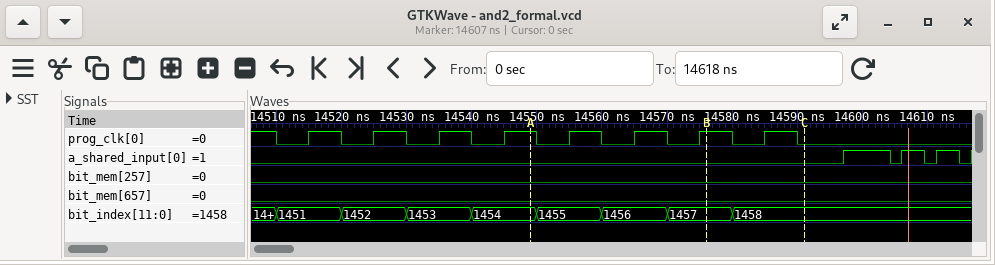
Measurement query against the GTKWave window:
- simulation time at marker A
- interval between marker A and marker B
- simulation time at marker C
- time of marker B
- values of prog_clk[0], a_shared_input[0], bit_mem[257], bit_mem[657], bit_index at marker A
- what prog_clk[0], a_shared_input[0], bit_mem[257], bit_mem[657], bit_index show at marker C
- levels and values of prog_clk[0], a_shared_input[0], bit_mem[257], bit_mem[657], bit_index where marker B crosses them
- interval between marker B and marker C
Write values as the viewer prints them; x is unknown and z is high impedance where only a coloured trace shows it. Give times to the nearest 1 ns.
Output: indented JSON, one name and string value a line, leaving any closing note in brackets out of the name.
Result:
{
  "simulation time at marker A": "14549 ns",
  "interval between marker A and marker B": "27 ns",
  "simulation time at marker C": "14591 ns",
  "time of marker B": "14576 ns",
  "values of prog_clk[0], a_shared_input[0], bit_mem[257], bit_mem[657], bit_index at marker A": "prog_clk[0]=1, a_shared_input[0]=0, bit_mem[257]=0, bit_mem[657]=0, bit_index=1454",
  "what prog_clk[0], a_shared_input[0], bit_mem[257], bit_mem[657], bit_index show at marker C": "prog_clk[0]=0, a_shared_input[0]=0, bit_mem[257]=0, bit_mem[657]=0, bit_index=1458",
  "levels and values of prog_clk[0], a_shared_input[0], bit_mem[257], bit_mem[657], bit_index where marker B crosses them": "prog_clk[0]=1, a_shared_input[0]=0, bit_mem[257]=0, bit_mem[657]=0, bit_index=1457",
  "interval between marker B and marker C": "15 ns"
}
